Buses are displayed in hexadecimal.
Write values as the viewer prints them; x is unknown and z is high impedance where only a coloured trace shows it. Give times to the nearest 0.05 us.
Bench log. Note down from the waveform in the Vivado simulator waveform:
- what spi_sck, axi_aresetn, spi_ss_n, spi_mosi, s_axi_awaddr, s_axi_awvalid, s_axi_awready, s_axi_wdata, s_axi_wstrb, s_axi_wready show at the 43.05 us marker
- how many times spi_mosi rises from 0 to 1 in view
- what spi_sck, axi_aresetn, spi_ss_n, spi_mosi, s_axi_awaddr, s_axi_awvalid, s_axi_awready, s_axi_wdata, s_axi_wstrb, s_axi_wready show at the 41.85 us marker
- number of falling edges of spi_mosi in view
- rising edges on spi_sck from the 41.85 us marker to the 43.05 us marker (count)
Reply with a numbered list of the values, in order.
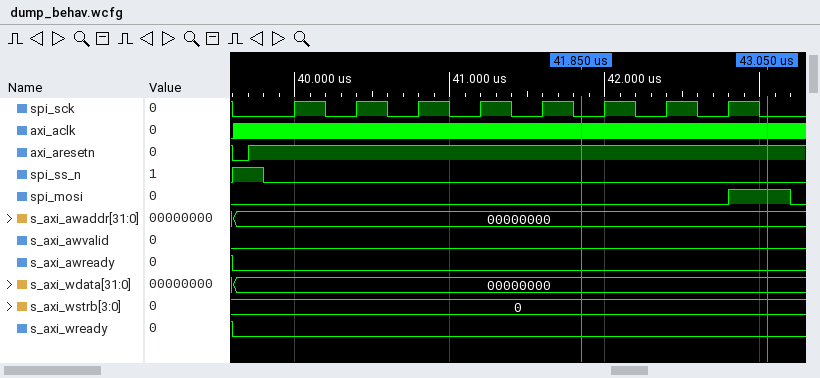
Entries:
1. spi_sck=0, axi_aresetn=1, spi_ss_n=0, spi_mosi=1, s_axi_awaddr=00000000, s_axi_awvalid=0, s_axi_awready=0, s_axi_wdata=00000000, s_axi_wstrb=0, s_axi_wready=0
2. 1
3. spi_sck=0, axi_aresetn=1, spi_ss_n=0, spi_mosi=0, s_axi_awaddr=00000000, s_axi_awvalid=0, s_axi_awready=0, s_axi_wdata=00000000, s_axi_wstrb=0, s_axi_wready=0
4. 1
5. 3
